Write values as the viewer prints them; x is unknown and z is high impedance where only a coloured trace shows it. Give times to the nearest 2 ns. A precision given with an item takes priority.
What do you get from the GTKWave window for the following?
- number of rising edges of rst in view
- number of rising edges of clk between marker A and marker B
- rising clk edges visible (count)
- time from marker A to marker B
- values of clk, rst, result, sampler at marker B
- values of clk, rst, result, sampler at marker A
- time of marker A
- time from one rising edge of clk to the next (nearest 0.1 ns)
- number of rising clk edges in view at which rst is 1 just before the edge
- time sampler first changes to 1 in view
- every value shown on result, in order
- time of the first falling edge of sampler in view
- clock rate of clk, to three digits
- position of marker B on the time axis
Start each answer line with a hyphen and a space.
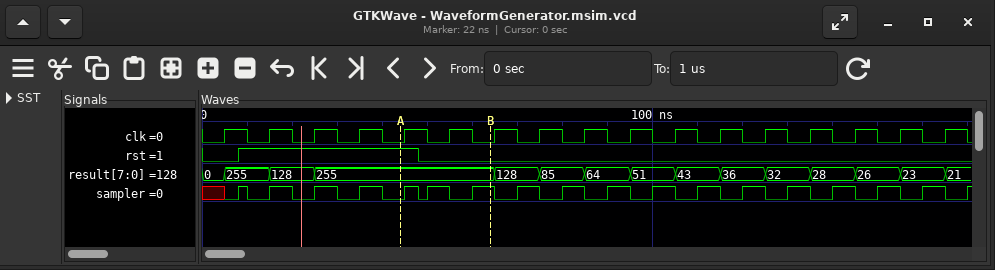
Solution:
- 1
- 2
- 17
- 20 ns
- clk=0, rst=0, result=255, sampler=1
- clk=0, rst=1, result=255, sampler=0
- 44 ns
- 10 ns
- 4
- 8 ns
- 0, 255, 128, 255, 128, 85, 64, 51, 43, 36, 32, 28, 26, 23, 21
- 10 ns
- 100 MHz
- 64 ns
